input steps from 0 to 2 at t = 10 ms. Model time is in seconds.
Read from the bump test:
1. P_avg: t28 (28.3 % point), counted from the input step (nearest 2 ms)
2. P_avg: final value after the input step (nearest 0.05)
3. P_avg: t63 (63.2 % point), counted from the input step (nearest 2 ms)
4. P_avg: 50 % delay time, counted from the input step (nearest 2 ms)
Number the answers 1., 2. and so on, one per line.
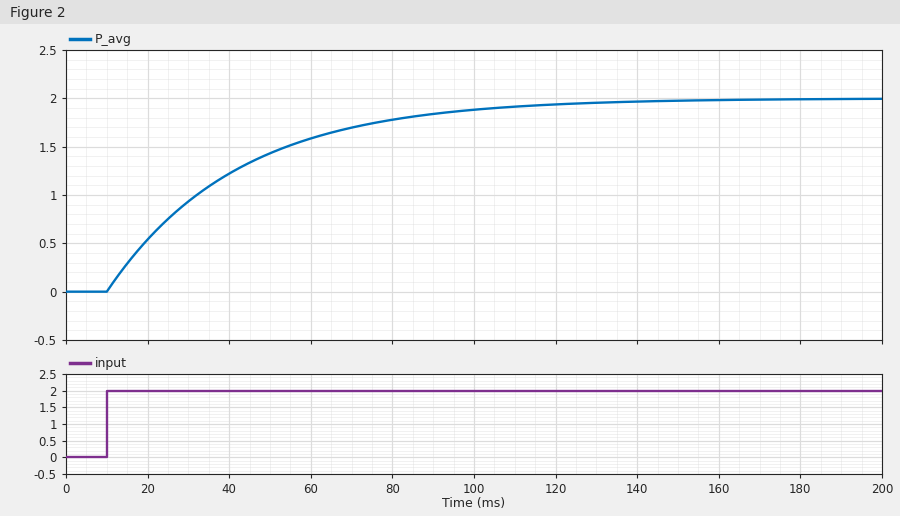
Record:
1. 10 ms
2. 2.00
3. 32 ms
4. 22 ms
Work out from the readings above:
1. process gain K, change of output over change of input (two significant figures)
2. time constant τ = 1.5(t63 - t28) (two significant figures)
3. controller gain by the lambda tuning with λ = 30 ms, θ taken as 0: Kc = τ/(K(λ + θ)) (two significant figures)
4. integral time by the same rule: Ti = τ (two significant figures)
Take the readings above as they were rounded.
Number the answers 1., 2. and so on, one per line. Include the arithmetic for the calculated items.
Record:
1. (2 - 0) / 2 = 1.0
2. 1.5 × (32 - 10) = 33 ms
3. 33 / (1 × (30 + 0)) = 1.1
4. 33 ms
